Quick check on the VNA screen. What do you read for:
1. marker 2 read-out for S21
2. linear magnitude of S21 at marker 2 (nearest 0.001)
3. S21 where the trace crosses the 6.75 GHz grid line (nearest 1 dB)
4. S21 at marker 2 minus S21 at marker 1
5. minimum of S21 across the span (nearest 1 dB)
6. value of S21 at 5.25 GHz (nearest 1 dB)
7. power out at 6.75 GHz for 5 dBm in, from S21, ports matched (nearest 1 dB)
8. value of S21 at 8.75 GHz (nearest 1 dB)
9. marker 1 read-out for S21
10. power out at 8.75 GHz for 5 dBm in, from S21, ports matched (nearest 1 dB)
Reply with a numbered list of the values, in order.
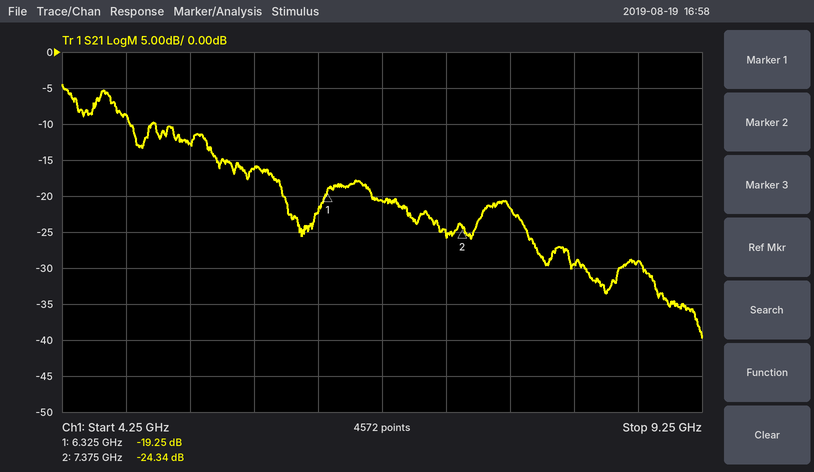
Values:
1. -24.34 dB
2. 0.061
3. -21 dB
4. -5.09 dB
5. -40 dB
6. -13 dB
7. -16 dBm
8. -29 dB
9. -19.25 dB
10. -24 dBm
